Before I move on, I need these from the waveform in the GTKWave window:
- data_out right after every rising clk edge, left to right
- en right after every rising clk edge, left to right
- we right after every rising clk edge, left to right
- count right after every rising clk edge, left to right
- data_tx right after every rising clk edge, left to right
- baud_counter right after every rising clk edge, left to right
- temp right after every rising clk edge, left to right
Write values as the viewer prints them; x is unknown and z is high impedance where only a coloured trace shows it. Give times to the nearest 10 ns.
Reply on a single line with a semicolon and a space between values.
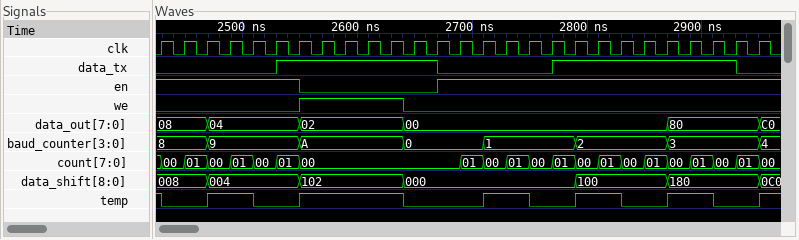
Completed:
08, 08, 04, 04, 04, 04, 02, 02, 02, 02, 02, 00, 00, 00, 00, 00, 00, 00, 00, 00, 00, 00, 80, 80, 80, 80, C0; 1 1 1 1 1 1 0 0 0 0 0 0 1 1 1 1 1 1 1 1 1 1 1 1 1 1 1; 0 0 0 0 0 0 1 1 1 1 1 0 0 0 0 0 0 0 0 0 0 0 0 0 0 0 0; 00, 01, 00, 01, 00, 01, 00, 00, 00, 00, 00, 00, 00, 01, 00, 01, 00, 01, 00, 01, 00, 01, 00, 01, 00, 01, 00; 0 0 0 0 0 1 1 1 1 1 1 1 0 0 0 0 0 1 1 1 1 1 1 1 1 0 0; 8, 8, 9, 9, 9, 9, A, A, A, A, A, 0, 0, 0, 1, 1, 1, 1, 2, 2, 2, 2, 3, 3, 3, 3, 4; 0 0 1 1 0 0 1 1 1 1 1 0 0 0 1 1 0 0 1 1 0 0 1 1 0 0 1
